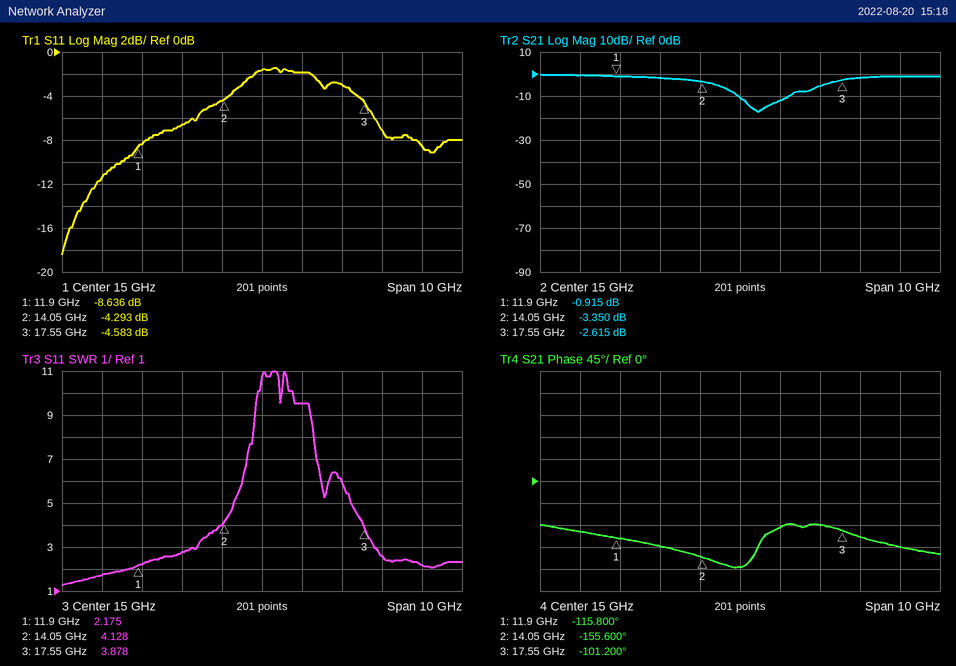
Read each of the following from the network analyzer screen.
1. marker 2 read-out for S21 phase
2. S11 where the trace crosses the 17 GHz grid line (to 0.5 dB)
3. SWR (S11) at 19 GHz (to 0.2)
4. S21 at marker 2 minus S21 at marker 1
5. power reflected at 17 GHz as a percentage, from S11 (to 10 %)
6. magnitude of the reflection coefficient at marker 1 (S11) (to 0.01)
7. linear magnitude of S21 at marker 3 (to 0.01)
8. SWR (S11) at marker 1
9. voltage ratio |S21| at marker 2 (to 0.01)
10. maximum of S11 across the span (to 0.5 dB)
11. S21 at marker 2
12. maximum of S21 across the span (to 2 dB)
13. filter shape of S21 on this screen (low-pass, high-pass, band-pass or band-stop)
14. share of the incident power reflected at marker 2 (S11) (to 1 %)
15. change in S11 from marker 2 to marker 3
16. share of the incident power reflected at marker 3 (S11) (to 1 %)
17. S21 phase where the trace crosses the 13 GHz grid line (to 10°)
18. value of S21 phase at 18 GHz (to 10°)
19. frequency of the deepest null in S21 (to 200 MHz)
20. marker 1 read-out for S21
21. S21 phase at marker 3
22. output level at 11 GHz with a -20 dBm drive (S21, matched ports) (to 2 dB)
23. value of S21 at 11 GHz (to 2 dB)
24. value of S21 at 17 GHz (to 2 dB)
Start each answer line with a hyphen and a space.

- -155.600°
- -3.0 dB
- 2.2
- -2.435 dB
- 50 %
- 0.37
- 0.74
- 2.175
- 0.68
- -1.5 dB
- -3.350 dB
- 0 dB
- band-stop
- 37 %
- -0.290 dB
- 35 %
- -130°
- -110°
- 15.4 GHz
- -0.915 dB
- -101.200°
- -20 dBm
- 0 dB
- -6 dB
